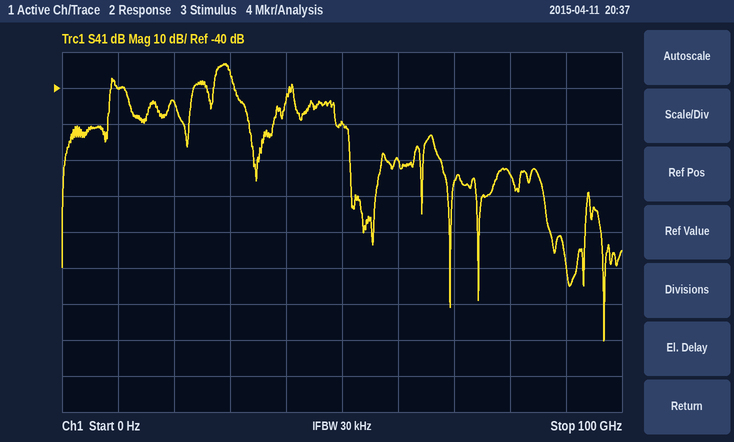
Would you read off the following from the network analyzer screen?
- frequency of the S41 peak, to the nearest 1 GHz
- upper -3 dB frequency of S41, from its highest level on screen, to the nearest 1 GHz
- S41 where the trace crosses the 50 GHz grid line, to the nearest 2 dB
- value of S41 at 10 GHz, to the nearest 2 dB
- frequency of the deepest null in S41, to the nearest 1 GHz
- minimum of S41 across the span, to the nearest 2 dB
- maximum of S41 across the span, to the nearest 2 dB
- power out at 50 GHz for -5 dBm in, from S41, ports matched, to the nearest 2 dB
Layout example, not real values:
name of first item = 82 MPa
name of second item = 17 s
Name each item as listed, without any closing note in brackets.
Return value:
frequency of the S41 peak, to the nearest 1 GHz = 29 GHz
upper -3 dB frequency of S41, from its highest level on screen, to the nearest 1 GHz = 30 GHz
S41 where the trace crosses the 50 GHz grid line, to the nearest 2 dB = -50 dB
value of S41 at 10 GHz, to the nearest 2 dB = -40 dB
frequency of the deepest null in S41, to the nearest 1 GHz = 97 GHz
minimum of S41 across the span, to the nearest 2 dB = -110 dB
maximum of S41 across the span, to the nearest 2 dB = -34 dB
power out at 50 GHz for -5 dBm in, from S41, ports matched, to the nearest 2 dB = -54 dBm
